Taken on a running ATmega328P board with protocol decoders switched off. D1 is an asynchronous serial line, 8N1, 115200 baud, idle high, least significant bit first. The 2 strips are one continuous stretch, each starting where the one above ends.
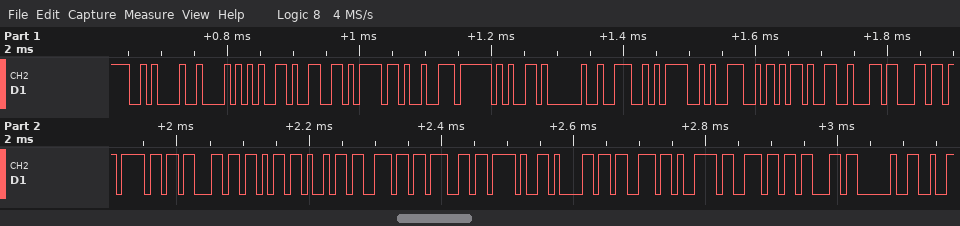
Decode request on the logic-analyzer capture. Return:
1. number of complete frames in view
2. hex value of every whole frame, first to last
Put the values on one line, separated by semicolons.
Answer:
27; 0A 42 65 66 6F 72 65 20 4E 4F 4E 2D 62 6C 6F 63 6B 69 6E 67 2F 61 73 79 6E 63 20
